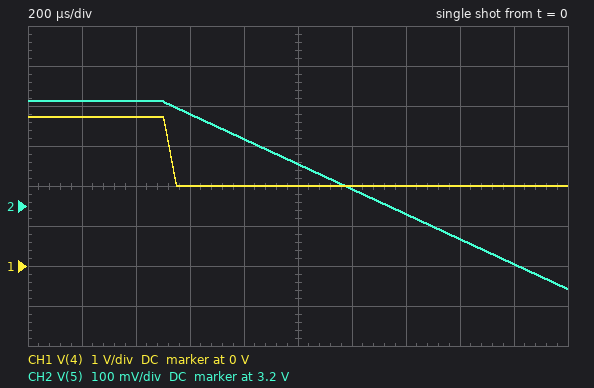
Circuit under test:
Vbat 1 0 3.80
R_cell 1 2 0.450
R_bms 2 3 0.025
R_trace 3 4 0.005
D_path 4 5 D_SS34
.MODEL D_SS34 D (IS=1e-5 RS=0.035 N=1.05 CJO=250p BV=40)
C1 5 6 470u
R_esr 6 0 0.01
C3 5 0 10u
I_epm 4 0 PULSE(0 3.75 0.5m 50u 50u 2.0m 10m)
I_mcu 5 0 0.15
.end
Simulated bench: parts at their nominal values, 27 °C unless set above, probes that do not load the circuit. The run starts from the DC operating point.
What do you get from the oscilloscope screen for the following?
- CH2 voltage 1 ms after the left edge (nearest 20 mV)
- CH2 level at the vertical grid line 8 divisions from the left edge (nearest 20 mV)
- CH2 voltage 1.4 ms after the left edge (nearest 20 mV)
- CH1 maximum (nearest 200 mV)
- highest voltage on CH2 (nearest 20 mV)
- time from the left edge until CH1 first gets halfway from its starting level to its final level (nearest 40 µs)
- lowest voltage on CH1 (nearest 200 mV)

3.30 V
3.12 V
3.18 V
3.8 V
3.46 V
520 µs
2.0 V
